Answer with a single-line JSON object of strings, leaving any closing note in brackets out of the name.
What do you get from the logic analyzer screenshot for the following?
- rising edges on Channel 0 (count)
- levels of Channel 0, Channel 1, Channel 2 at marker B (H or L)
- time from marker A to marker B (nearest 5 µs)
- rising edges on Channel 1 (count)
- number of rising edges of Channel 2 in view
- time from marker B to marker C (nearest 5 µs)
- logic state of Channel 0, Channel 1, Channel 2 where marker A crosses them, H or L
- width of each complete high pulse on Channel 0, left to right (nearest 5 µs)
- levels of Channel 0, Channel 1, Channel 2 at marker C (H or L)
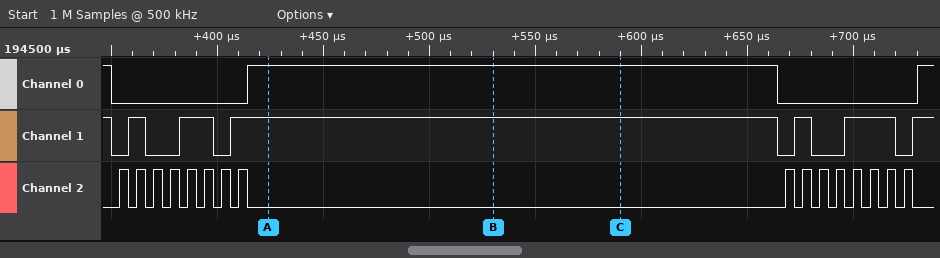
{"rising edges on Channel 0": "2", "levels of Channel 0, Channel 1, Channel 2 at marker B": "Channel 0=H, Channel 1=H, Channel 2=L", "time from marker A to marker B": "105 µs", "rising edges on Channel 1": "6", "number of rising edges of Channel 2 in view": "16", "time from marker B to marker C": "60 µs", "logic state of Channel 0, Channel 1, Channel 2 where marker A crosses them, H or L": "Channel 0=H, Channel 1=H, Channel 2=L", "width of each complete high pulse on Channel 0, left to right": "250 µs", "levels of Channel 0, Channel 1, Channel 2 at marker C": "Channel 0=H, Channel 1=H, Channel 2=L"}
